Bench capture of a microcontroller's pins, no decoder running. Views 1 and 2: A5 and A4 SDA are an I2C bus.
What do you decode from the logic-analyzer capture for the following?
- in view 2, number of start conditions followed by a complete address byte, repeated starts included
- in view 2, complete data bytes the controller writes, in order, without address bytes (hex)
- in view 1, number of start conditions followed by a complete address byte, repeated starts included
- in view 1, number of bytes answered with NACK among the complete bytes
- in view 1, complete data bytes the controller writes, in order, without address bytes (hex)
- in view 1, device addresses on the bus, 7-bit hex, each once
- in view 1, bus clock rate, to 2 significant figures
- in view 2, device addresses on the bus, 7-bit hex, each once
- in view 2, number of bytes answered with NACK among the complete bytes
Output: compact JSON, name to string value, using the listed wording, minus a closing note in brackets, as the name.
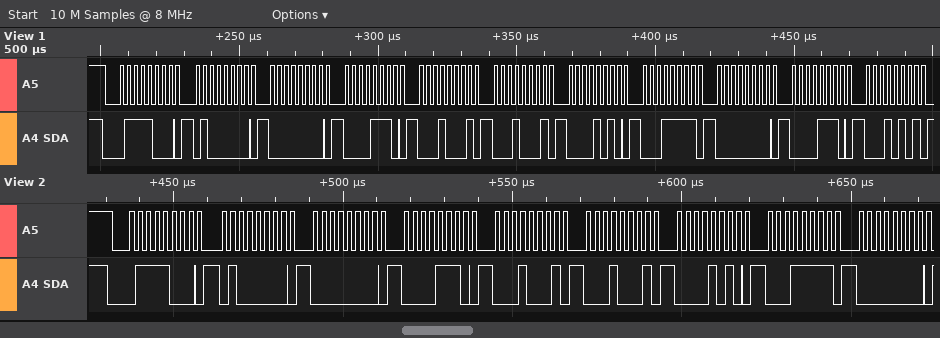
{"in view 2, number of start conditions followed by a complete address byte, repeated starts included": "1", "in view 2, complete data bytes the controller writes, in order, without address bytes": "40 00 0E 11 11 0A 1F 00", "in view 1, number of start conditions followed by a complete address byte, repeated starts included": "1", "in view 1, number of bytes answered with NACK among the complete bytes": "0", "in view 1, complete data bytes the controller writes, in order, without address bytes": "40 00 0E 11 11 0A 1F 00 0E 15", "in view 1, device addresses on the bus, 7-bit hex, each once": "0x3C", "in view 1, bus clock rate, to 2 significant figures": "400 kHz", "in view 2, device addresses on the bus, 7-bit hex, each once": "0x3C", "in view 2, number of bytes answered with NACK among the complete bytes": "0"}
